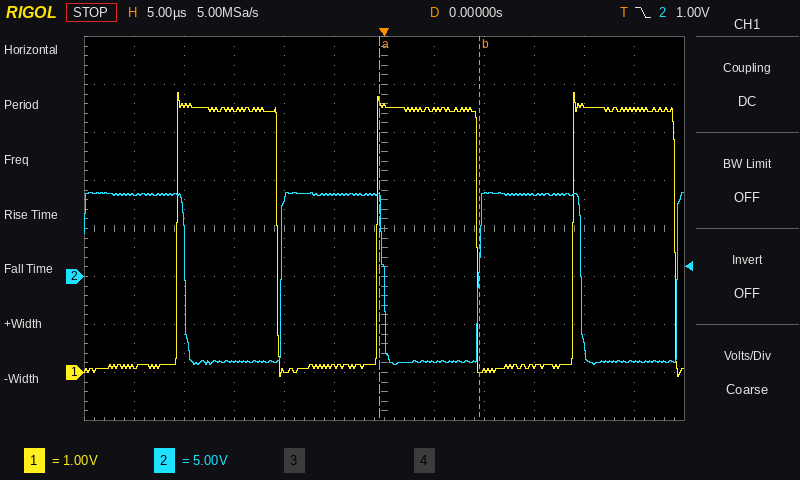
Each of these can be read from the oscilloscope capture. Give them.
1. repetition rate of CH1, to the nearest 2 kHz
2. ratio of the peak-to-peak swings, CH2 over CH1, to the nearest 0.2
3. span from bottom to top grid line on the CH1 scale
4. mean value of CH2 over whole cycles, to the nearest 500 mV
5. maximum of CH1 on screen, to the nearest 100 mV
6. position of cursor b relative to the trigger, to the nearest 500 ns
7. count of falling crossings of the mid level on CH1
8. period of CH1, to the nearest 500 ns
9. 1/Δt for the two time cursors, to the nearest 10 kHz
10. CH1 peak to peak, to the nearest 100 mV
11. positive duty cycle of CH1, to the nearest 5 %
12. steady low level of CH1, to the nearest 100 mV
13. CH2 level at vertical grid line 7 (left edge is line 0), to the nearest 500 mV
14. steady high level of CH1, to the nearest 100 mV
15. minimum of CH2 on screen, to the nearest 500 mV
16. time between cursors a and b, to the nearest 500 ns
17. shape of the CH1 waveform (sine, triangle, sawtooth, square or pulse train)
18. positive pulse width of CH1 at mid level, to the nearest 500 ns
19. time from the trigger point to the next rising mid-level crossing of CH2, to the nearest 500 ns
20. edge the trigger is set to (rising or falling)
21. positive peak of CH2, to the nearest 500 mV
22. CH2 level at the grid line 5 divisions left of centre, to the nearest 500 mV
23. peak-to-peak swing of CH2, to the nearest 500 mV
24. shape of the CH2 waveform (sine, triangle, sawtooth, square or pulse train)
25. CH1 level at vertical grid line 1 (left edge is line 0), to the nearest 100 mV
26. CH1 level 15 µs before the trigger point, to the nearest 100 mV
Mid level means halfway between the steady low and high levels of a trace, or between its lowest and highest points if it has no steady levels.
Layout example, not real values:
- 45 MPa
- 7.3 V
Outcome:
- 50 kHz
- 3.0
- 8 V
- 0.0 V
- 5.8 V
- +9.5 µs
- 3
- 20.0 µs
- 100 kHz
- 5.9 V
- 50 %
- 100 mV
- -9.0 V
- 5.5 V
- -9.0 V
- 10.0 µs
- square
- 10.0 µs
- 9.5 µs
- falling
- 9.0 V
- 8.5 V
- 18.0 V
- square
- 100 mV
- 5.5 V
